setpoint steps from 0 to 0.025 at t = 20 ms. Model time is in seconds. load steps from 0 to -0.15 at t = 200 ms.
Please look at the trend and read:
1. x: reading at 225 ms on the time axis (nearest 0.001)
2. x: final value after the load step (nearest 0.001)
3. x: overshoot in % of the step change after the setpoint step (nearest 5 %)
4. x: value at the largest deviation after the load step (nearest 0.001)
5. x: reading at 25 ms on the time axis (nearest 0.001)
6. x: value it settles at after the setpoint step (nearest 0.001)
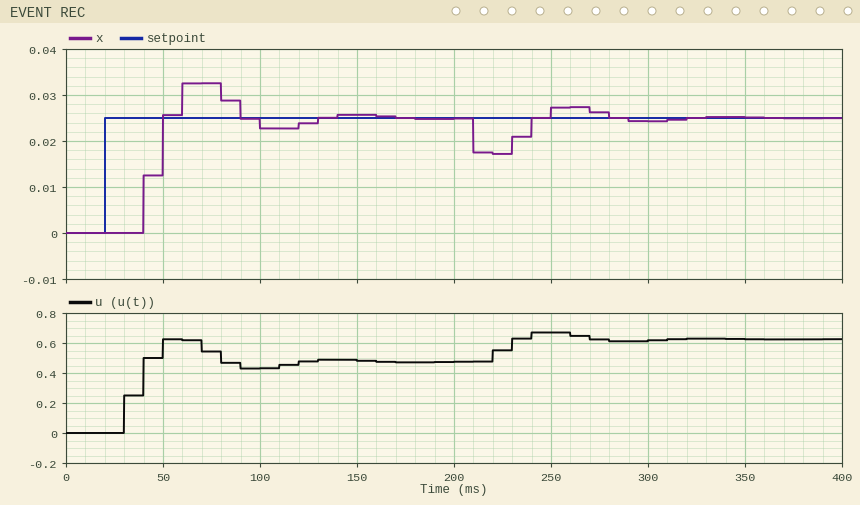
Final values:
0.017
0.025
30 %
0.017
0.000
0.025
